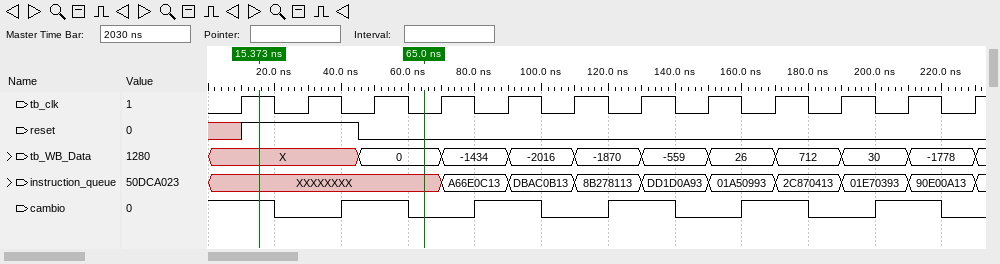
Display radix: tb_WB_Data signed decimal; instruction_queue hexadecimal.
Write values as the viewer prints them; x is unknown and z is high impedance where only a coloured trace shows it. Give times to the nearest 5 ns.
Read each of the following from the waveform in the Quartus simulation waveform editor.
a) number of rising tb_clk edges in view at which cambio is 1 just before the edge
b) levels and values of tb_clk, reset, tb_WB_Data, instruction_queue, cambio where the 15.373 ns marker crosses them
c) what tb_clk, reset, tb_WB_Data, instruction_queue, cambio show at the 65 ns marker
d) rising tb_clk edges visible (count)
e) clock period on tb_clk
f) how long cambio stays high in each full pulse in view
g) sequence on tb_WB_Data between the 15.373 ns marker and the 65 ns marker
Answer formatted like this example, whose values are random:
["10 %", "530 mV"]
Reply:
["6", "tb_clk=1, reset=1, tb_WB_Data=X, instruction_queue=XXXXXXXX, cambio=1", "tb_clk=0, reset=0, tb_WB_Data=0, instruction_queue=XXXXXXXX, cambio=0", "12", "20 ns", "20 ns, 20 ns, 20 ns, 20 ns, 20 ns", "X, 0"]
